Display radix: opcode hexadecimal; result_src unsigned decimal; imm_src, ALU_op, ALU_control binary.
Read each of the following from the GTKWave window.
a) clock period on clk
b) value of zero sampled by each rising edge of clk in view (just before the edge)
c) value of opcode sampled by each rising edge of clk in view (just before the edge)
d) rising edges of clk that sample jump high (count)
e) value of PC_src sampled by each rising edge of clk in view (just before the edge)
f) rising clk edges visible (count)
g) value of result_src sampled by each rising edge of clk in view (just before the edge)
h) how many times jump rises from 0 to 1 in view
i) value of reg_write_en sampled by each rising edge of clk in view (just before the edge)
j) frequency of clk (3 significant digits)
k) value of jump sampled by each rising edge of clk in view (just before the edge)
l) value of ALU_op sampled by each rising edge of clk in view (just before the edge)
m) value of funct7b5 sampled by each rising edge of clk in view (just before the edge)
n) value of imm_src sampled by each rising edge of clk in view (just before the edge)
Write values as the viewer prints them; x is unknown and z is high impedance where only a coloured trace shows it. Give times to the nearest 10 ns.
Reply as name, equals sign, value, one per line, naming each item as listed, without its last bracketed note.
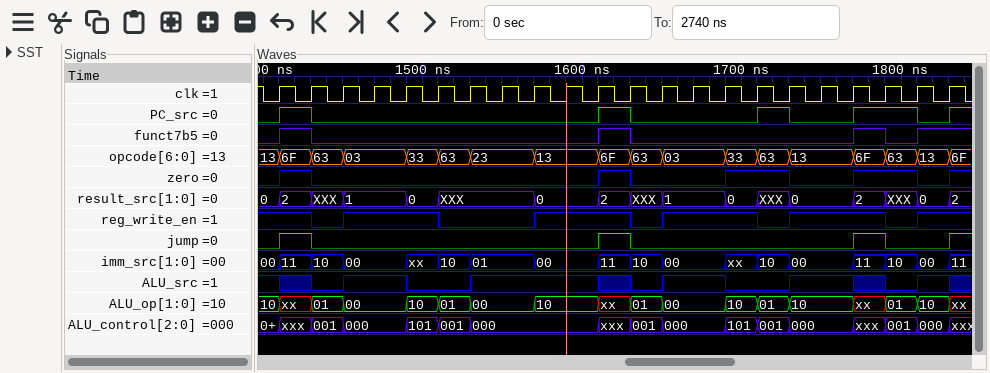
clock period on clk = 20 ns
value of zero sampled by each rising edge of clk in view = 0 1 0 0 0 0 0 0 0 0 0 1 0 0 0 1 1 0 0 1 1 0
value of opcode sampled by each rising edge of clk in view = 13, 6F, 63, 03, 03, 33, 63, 23, 23, 13, 13, 6F, 63, 03, 03, 33, 63, 13, 13, 6F, 63, 13
rising edges of clk that sample jump high = 3
value of PC_src sampled by each rising edge of clk in view = 0 1 0 0 0 0 0 0 0 0 0 1 0 0 0 0 1 0 0 1 1 0
rising clk edges visible = 22
value of result_src sampled by each rising edge of clk in view = 0, 2, XXX, 1, 1, 0, XXX, XXX, XXX, 0, 0, 2, XXX, 1, 1, 0, XXX, 0, 0, 2, XXX, 0
how many times jump rises from 0 to 1 in view = 4
value of reg_write_en sampled by each rising edge of clk in view = 1 1 0 1 1 1 0 0 0 1 1 1 0 1 1 1 0 1 1 1 0 1
frequency of clk = 50.0 MHz
value of jump sampled by each rising edge of clk in view = 0 1 0 0 0 0 0 0 0 0 0 1 0 0 0 0 0 0 0 1 0 0
value of ALU_op sampled by each rising edge of clk in view = 10, xx, 01, 00, 00, 10, 01, 00, 00, 10, 10, xx, 01, 00, 00, 10, 01, 10, 10, xx, 01, 10
value of funct7b5 sampled by each rising edge of clk in view = 0 1 0 0 0 0 0 0 0 0 0 1 0 0 0 0 0 0 0 1 0 1
value of imm_src sampled by each rising edge of clk in view = 00, 11, 10, 00, 00, xx, 10, 01, 01, 00, 00, 11, 10, 00, 00, xx, 10, 00, 00, 11, 10, 00
